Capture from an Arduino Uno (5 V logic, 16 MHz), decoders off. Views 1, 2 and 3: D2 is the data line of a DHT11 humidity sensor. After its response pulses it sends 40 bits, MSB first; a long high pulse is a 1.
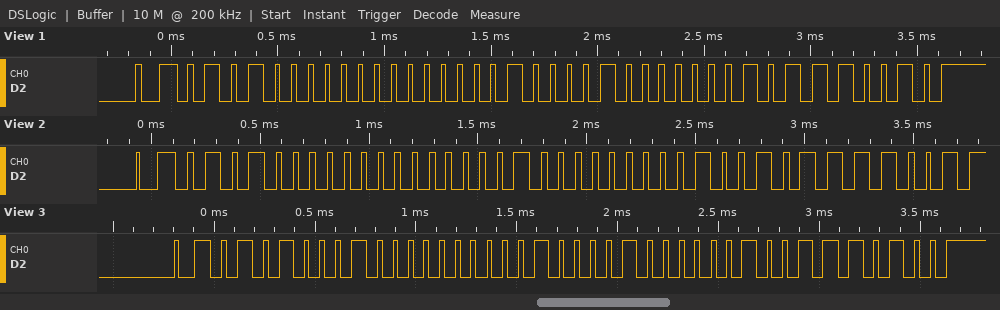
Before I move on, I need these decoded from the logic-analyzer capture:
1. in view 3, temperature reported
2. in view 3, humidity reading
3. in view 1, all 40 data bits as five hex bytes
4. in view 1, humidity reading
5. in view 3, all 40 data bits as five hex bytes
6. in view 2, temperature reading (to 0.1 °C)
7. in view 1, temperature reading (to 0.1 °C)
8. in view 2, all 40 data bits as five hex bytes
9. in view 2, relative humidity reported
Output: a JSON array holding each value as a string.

["33.2 °C", "81 %", "50 00 21 01 72", "80 %", "51 00 21 02 74", "32.9 °C", "33.1 °C", "50 00 20 09 79", "80 %"]
